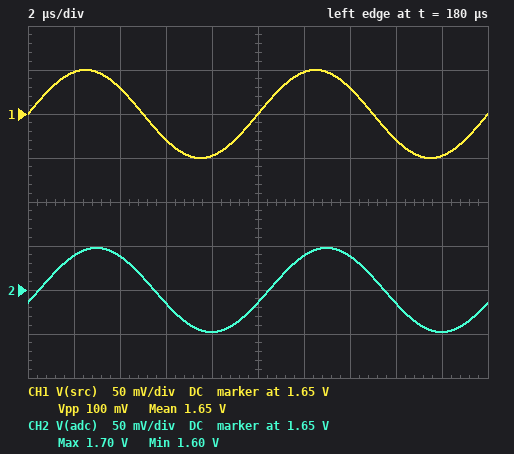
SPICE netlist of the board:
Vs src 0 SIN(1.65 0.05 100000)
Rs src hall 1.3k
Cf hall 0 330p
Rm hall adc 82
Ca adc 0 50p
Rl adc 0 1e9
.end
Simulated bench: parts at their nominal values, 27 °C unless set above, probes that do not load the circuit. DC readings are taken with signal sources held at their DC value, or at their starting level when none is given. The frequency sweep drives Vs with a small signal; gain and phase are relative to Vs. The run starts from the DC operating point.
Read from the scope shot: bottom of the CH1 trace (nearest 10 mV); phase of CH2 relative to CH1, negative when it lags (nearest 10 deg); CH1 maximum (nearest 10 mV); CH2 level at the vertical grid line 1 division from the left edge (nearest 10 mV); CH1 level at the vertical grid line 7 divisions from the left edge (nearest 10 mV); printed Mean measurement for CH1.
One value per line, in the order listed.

1.60 V
-20 deg
1.70 V
1.69 V
1.68 V
1.65 V
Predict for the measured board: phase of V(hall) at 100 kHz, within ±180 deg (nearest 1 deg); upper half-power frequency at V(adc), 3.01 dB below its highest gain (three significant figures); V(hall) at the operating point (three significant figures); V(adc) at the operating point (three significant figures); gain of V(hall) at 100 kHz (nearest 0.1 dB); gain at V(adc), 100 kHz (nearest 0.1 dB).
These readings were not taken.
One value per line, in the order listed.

-17 deg
322 kHz
1.65 V
1.65 V
-0.4 dB
-0.4 dB
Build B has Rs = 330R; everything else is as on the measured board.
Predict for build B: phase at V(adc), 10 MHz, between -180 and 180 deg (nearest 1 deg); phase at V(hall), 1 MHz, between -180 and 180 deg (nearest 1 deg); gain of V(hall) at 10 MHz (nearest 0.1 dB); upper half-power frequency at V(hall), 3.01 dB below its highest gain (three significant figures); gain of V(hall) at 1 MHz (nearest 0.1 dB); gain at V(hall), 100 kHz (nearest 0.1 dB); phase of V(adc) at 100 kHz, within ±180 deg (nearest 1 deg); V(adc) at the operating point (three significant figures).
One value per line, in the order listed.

-95 deg
-38 deg
-18.0 dB
1.26 MHz
-2.1 dB
0 dB
-5 deg
1.65 V
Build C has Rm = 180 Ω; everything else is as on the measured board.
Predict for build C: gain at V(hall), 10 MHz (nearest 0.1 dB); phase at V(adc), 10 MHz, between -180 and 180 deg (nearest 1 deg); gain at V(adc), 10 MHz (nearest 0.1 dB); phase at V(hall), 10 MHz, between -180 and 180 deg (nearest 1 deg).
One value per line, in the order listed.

-29.6 dB
-114 deg
-30.8 dB
-85 deg
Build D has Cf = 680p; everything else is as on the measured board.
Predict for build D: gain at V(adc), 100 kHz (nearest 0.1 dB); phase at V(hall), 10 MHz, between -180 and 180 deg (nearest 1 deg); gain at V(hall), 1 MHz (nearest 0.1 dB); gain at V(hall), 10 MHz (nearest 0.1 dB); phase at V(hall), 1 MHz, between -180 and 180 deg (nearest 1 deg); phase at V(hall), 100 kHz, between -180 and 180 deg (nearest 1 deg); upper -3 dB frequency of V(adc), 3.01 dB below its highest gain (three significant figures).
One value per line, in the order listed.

-1.3 dB
-88 deg
-15.6 dB
-35.5 dB
-80 deg
-31 deg
168 kHz
